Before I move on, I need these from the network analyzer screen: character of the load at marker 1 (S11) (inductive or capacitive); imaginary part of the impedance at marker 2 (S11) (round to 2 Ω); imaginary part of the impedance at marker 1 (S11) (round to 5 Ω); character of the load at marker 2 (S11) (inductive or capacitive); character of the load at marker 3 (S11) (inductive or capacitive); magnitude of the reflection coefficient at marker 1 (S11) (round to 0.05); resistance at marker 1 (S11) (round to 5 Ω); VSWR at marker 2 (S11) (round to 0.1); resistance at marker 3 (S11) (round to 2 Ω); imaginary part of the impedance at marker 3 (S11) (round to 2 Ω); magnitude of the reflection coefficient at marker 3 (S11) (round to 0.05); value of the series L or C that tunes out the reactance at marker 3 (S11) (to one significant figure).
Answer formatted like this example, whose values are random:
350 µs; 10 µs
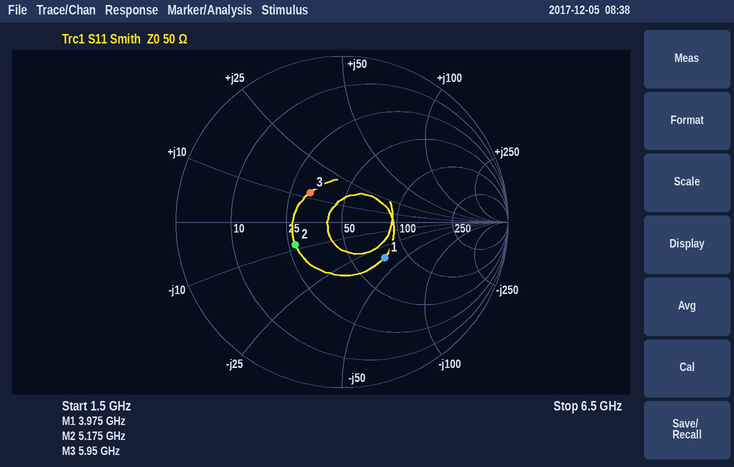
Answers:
capacitive; -8 Ω; -35 Ω; capacitive; inductive; 0.35; 75 Ω; 1.9; 32 Ω; +12 Ω; 0.25; 2 pF
